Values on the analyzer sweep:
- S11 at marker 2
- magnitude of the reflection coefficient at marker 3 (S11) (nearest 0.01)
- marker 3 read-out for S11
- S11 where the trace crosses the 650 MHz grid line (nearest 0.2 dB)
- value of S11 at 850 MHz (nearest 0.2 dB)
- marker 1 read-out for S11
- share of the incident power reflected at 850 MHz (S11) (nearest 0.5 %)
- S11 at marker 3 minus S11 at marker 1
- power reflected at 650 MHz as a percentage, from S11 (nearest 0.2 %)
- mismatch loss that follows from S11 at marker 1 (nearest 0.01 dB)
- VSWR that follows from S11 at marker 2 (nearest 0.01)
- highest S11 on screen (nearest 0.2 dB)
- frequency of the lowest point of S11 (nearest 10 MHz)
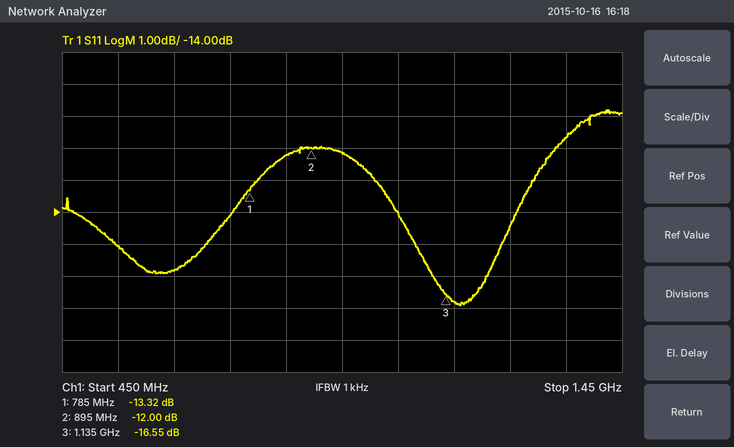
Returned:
-12.00 dB
0.15
-16.55 dB
-15.8 dB
-12.2 dB
-13.32 dB
6.0 %
-3.23 dB
2.6 %
0.21 dB
1.67
-10.8 dB
1.16 GHz
